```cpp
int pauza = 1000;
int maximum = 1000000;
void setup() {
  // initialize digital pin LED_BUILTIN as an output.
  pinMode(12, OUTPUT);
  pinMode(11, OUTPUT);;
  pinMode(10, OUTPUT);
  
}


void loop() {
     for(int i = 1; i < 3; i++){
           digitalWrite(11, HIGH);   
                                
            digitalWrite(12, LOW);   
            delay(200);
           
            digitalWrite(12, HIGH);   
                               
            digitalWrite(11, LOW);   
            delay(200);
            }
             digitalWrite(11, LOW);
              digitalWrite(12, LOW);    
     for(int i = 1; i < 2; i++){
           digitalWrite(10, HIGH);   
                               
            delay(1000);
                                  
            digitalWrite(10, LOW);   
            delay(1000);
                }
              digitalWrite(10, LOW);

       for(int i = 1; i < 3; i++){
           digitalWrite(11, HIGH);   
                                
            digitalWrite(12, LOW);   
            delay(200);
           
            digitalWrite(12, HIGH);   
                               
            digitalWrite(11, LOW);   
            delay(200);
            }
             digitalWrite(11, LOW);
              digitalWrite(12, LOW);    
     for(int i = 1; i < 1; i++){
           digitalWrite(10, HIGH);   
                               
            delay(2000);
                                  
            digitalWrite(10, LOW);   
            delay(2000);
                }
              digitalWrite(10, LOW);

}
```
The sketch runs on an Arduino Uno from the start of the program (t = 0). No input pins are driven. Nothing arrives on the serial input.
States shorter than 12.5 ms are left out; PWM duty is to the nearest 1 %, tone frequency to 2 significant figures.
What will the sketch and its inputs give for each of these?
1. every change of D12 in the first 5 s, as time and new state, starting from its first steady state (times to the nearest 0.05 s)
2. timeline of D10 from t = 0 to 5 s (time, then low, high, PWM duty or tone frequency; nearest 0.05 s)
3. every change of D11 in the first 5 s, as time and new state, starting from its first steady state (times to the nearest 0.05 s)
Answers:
0 s low; 0.2 s high; 0.4 s low; 0.6 s high; 0.8 s low; 3 s high; 3.2 s low; 3.4 s high; 3.6 s low; 3.8 s high; 4 s low; 4.2 s high; 4.4 s low
0 s low; 0.8 s high; 1.8 s low; 4.4 s high
0 s high; 0.2 s low; 0.4 s high; 0.6 s low; 2.8 s high; 3 s low; 3.2 s high; 3.4 s low; 3.6 s high; 3.8 s low; 4 s high; 4.2 s low
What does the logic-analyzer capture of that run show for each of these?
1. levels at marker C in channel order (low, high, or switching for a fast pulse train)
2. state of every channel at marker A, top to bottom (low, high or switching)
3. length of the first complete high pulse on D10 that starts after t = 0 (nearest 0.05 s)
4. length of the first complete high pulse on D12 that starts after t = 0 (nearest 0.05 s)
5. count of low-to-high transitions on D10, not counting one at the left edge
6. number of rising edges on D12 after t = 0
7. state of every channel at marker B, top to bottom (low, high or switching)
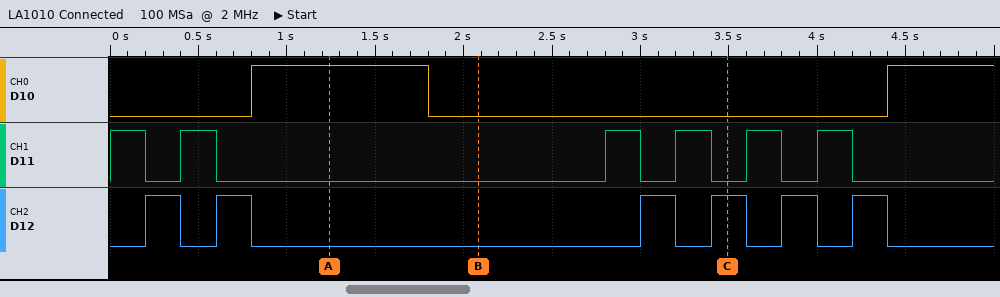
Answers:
D10 low, D11 low, D12 high
D10 high, D11 low, D12 low
1.00 s
0.20 s
2
6
D10 low, D11 low, D12 low
